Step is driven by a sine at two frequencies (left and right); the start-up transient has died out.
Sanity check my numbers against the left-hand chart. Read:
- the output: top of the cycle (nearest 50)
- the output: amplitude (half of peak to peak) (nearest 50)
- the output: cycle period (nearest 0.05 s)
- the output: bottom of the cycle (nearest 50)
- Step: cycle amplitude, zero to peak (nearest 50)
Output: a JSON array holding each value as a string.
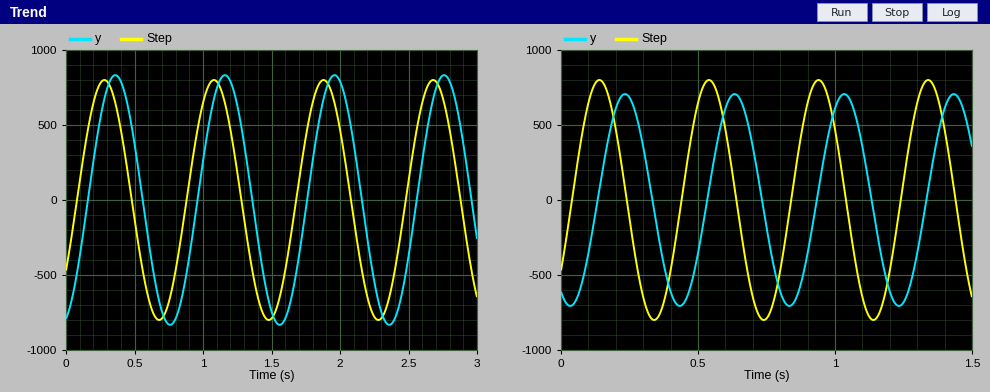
["850", "850", "0.80 s", "-850", "800"]
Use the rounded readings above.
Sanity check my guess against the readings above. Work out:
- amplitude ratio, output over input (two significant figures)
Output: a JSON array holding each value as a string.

["1.1"]
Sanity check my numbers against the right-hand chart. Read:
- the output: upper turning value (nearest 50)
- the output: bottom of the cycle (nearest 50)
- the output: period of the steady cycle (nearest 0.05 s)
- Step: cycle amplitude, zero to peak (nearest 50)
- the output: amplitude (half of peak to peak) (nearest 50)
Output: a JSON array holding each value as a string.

["700", "-700", "0.40 s", "800", "700"]
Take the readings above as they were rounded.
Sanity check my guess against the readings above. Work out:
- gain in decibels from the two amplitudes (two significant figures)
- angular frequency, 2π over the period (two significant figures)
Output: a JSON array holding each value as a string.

["-1.2 dB", "16 rad/s"]
